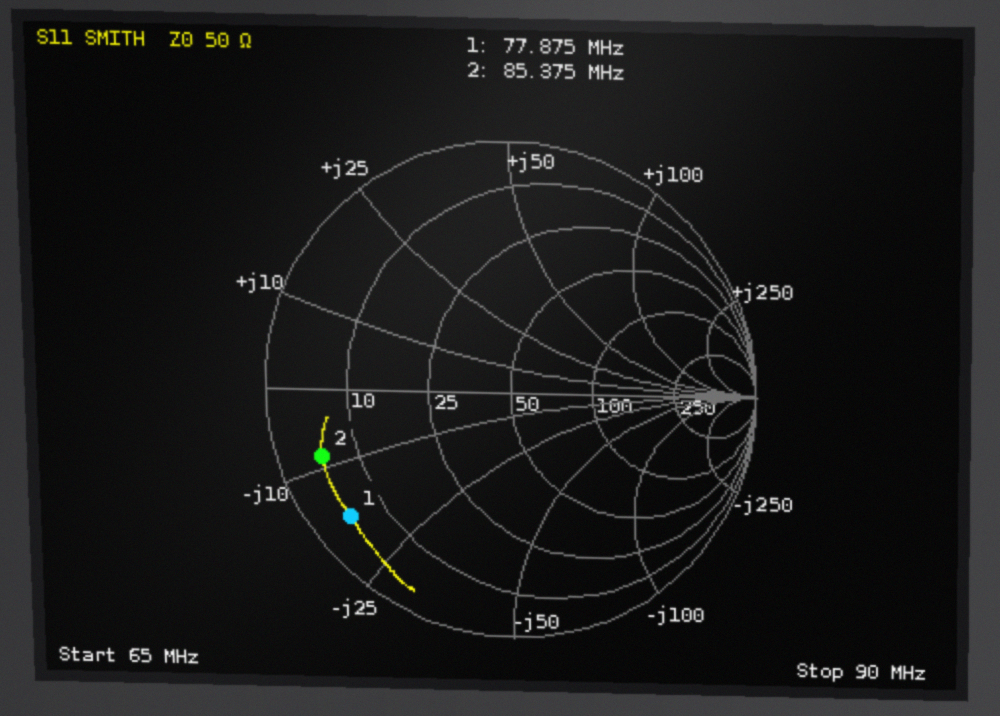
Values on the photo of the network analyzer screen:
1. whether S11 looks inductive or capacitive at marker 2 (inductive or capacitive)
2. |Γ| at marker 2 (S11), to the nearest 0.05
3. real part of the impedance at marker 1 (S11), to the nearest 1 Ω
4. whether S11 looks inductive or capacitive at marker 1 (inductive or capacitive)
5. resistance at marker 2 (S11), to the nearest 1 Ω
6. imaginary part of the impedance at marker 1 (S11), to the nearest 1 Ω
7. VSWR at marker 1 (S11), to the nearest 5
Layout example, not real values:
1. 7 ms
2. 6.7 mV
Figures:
1. capacitive
2. 0.80
3. 5 Ω
4. capacitive
5. 5 Ω
6. -17 Ω
7. 10
